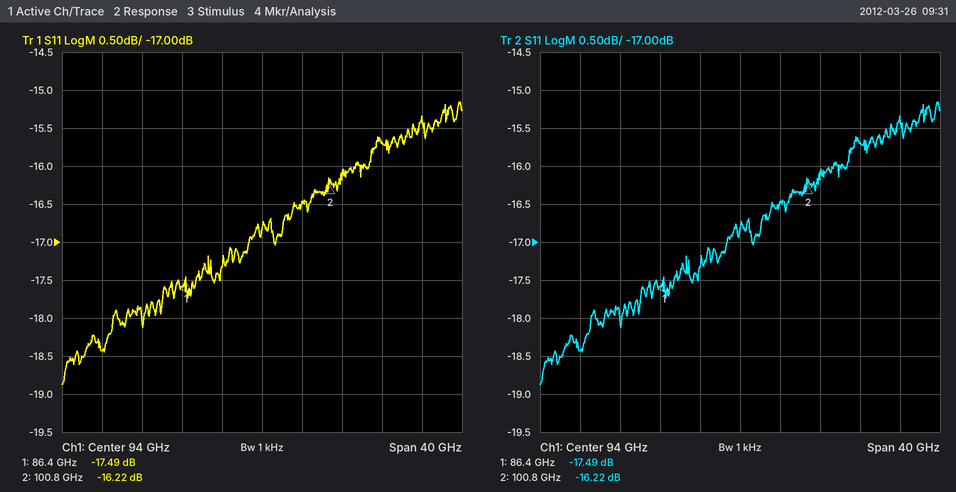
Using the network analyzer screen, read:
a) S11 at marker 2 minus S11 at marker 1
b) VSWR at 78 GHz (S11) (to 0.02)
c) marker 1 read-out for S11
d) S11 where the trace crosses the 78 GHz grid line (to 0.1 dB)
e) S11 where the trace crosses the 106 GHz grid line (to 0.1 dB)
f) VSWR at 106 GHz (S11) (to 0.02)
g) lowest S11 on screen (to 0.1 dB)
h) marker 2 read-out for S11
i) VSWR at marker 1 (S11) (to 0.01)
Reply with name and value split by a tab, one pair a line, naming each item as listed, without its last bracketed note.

S11 at marker 2 minus S11 at marker 1	1.27 dB
VSWR at 78 GHz (S11)	1.28
marker 1 read-out for S11	-17.49 dB
S11 where the trace crosses the 78 GHz grid line	-18.4 dB
S11 where the trace crosses the 106 GHz grid line	-15.7 dB
VSWR at 106 GHz (S11)	1.40
lowest S11 on screen	-18.9 dB
marker 2 read-out for S11	-16.22 dB
VSWR at marker 1 (S11)	1.31
